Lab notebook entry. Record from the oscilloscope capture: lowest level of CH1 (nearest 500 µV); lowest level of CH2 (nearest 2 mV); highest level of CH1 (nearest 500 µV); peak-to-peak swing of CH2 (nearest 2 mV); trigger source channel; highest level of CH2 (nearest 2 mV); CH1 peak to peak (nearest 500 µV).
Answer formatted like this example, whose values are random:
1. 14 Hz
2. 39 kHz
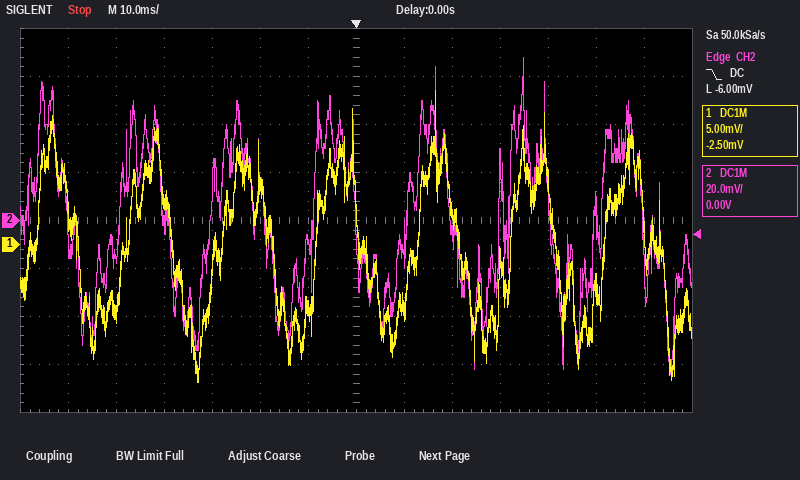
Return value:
1. -14.5 mV
2. -64 mV
3. 16.0 mV
4. 132 mV
5. CH2
6. 68 mV
7. 30.5 mV
